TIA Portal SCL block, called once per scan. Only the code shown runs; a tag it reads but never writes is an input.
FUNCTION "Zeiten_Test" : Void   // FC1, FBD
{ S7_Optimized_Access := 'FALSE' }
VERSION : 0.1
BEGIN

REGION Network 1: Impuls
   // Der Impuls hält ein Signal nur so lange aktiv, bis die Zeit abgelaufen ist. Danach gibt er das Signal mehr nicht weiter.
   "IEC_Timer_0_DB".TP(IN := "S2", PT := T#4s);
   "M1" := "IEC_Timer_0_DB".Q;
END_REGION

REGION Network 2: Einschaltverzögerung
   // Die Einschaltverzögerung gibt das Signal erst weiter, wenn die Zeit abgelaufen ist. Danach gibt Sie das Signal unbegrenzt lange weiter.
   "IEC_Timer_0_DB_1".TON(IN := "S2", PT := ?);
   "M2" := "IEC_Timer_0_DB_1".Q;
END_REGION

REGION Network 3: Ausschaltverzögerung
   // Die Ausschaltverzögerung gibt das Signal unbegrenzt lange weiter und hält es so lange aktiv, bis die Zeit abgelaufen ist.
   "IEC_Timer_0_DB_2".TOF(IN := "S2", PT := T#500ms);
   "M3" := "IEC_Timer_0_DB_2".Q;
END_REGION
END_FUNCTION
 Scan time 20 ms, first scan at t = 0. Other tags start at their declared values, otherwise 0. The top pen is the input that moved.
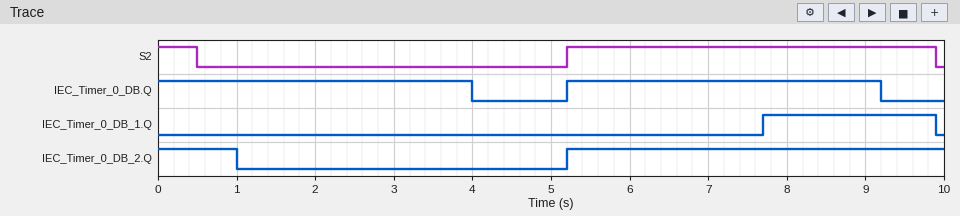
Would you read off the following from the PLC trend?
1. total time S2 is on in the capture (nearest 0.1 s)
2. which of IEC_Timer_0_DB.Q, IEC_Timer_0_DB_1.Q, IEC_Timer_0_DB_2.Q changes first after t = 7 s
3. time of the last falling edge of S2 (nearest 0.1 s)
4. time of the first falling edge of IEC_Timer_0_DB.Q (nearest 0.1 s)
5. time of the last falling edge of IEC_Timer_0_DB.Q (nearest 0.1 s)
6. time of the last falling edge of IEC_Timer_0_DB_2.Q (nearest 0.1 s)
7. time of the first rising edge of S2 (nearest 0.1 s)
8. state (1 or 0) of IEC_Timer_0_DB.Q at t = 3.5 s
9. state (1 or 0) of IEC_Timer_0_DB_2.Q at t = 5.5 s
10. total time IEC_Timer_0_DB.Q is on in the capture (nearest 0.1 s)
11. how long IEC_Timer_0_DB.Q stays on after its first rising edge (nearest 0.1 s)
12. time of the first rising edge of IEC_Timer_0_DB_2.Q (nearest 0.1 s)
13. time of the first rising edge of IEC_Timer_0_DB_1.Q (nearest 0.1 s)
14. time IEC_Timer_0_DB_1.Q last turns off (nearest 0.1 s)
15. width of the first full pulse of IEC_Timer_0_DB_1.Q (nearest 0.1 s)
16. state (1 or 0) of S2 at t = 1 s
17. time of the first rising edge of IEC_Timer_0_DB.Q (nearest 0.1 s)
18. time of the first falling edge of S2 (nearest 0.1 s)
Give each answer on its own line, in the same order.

5.2 s
IEC_Timer_0_DB_1.Q
9.9 s
4.0 s
9.2 s
1.0 s
5.2 s
1
1
8.0 s
4.0 s
5.2 s
7.7 s
9.9 s
2.2 s
0
5.2 s
0.5 s
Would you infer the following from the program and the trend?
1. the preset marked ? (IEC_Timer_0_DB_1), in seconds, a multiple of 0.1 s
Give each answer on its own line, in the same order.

2.5 s
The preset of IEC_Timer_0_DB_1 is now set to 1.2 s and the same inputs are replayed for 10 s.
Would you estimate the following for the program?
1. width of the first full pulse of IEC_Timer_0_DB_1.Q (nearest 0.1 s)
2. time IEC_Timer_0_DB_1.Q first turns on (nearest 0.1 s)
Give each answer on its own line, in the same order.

3.5 s
6.4 s
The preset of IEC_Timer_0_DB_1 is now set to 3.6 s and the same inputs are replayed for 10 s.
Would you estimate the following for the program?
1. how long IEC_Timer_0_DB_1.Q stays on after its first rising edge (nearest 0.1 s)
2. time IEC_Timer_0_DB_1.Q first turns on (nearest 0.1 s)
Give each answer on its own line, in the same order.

1.1 s
8.8 s
